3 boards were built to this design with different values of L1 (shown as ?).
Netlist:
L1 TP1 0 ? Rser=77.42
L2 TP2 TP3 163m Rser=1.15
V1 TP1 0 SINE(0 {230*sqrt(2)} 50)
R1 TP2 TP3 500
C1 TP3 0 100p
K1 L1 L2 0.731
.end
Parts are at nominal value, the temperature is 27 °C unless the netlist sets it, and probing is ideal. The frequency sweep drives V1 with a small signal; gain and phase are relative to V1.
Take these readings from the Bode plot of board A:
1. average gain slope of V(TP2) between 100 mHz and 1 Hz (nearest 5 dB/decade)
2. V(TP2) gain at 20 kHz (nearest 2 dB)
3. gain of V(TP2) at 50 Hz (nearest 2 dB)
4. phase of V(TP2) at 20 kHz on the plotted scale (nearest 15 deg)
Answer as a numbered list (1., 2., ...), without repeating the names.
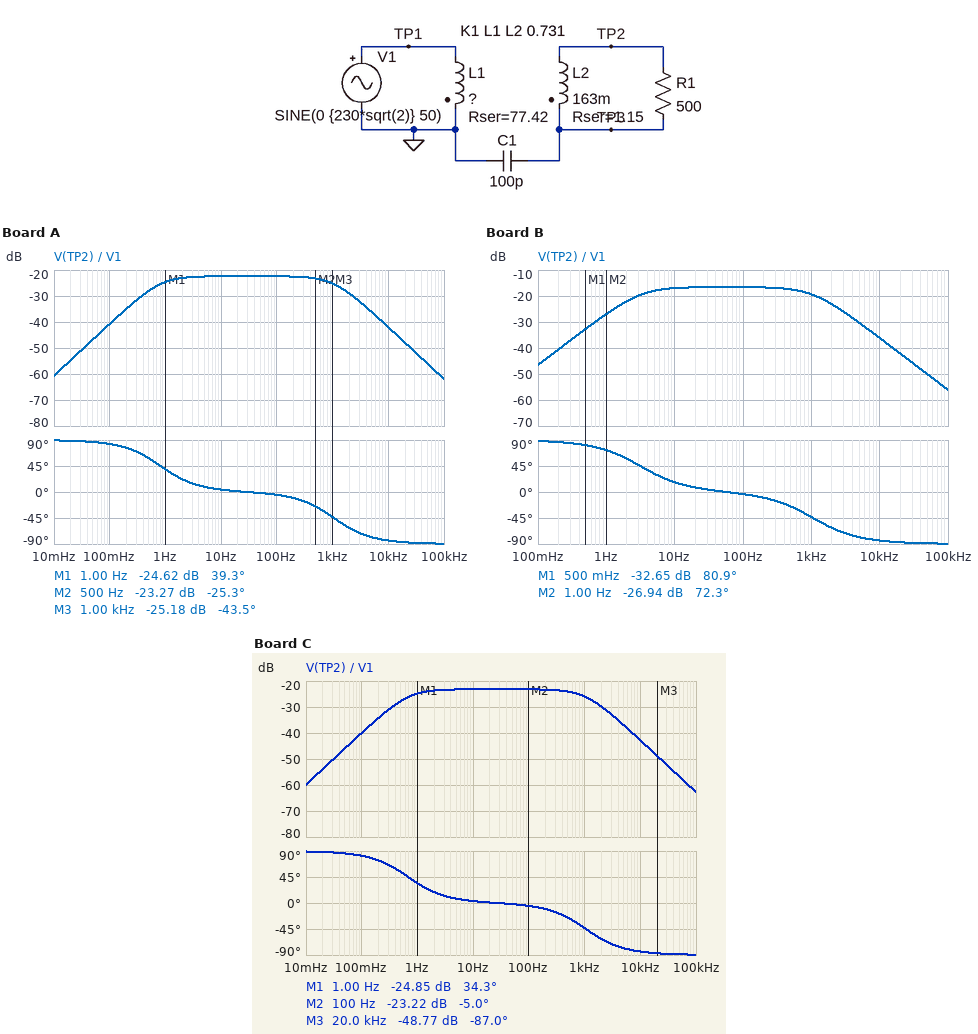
1. 15 dB/decade
2. -48 dB
3. -22 dB
4. -90 deg
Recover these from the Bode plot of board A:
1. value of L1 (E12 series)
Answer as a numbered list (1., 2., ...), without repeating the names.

1. 15 H
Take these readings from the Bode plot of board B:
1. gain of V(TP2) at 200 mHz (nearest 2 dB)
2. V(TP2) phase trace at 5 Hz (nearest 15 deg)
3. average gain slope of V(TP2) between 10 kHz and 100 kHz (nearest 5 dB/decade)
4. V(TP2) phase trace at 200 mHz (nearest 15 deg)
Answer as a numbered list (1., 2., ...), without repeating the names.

1. -40 dB
2. 30 deg
3. -20 dB/decade
4. 90 deg
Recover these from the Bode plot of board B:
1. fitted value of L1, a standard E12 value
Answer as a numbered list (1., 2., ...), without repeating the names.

1. 3.9 H
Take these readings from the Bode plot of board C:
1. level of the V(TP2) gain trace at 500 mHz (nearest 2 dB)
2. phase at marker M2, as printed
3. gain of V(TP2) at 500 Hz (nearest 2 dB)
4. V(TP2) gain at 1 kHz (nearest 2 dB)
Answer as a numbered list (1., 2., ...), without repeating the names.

1. -28 dB
2. -5.0 deg
3. -24 dB
4. -26 dB
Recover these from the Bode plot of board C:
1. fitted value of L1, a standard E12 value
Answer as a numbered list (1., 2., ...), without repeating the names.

1. 18 H
